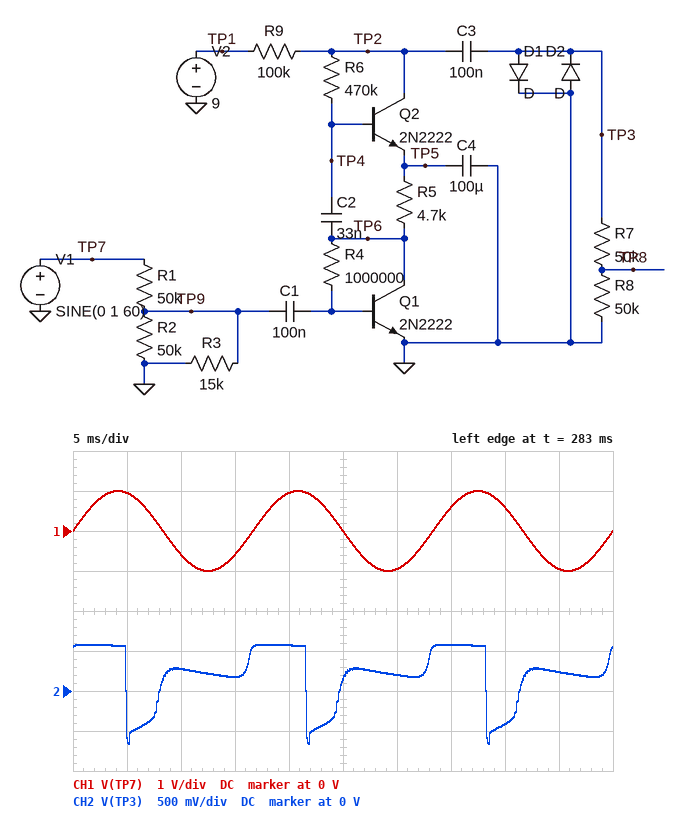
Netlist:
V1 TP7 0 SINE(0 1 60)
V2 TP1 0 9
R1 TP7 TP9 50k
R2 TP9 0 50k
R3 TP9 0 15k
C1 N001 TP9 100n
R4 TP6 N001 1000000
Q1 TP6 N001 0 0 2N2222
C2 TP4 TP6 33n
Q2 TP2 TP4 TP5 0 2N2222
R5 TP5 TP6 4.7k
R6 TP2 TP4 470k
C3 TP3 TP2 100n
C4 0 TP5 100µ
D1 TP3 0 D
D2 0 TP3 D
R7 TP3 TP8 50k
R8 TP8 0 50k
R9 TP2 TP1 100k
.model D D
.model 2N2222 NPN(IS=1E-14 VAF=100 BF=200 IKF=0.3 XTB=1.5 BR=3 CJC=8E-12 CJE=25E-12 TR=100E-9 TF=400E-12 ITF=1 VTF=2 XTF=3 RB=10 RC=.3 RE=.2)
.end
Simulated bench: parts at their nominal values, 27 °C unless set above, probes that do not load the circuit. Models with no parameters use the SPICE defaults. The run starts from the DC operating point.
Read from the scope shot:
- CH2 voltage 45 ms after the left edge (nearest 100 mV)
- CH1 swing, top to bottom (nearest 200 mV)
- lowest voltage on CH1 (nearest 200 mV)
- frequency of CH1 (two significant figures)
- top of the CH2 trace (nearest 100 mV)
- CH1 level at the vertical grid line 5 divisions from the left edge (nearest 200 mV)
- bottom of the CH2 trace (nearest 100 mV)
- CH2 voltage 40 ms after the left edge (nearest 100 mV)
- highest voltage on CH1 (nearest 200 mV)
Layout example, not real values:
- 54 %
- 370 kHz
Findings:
- 200 mV
- 2.0 V
- -1.0 V
- 60 Hz
- 600 mV
- 0 V
- -700 mV
- -400 mV
- 1.0 V
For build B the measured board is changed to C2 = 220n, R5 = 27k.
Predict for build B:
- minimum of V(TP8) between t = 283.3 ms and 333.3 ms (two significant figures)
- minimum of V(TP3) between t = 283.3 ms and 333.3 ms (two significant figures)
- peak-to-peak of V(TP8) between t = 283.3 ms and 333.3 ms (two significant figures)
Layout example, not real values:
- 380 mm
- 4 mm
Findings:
- -320 mV
- -640 mV
- 610 mV
